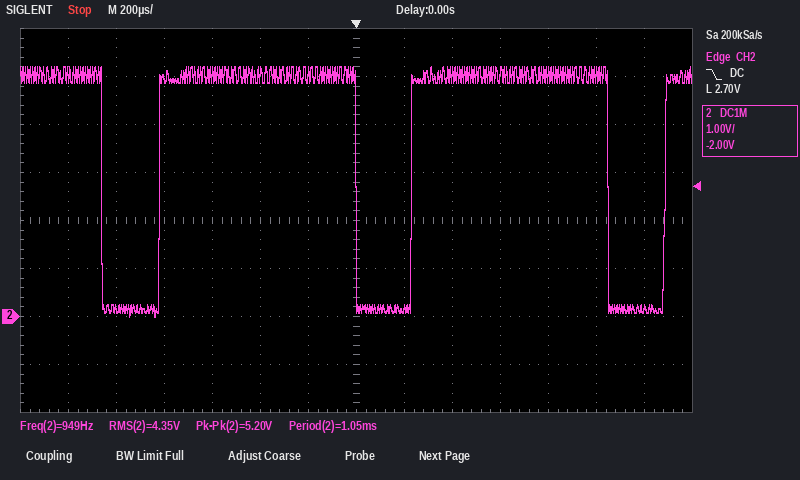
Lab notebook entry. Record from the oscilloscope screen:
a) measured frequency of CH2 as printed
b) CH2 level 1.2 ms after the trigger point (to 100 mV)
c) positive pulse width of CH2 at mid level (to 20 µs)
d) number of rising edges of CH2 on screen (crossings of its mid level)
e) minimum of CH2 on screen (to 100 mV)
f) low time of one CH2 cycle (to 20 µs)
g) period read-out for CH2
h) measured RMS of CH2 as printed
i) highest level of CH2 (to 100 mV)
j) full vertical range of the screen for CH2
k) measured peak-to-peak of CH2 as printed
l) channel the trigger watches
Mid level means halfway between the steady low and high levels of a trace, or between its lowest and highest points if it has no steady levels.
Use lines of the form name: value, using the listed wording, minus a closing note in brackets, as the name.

measured frequency of CH2 as printed: 949 Hz
CH2 level 1.2 ms after the trigger point: 200 mV
positive pulse width of CH2 at mid level: 820 µs
number of rising edges of CH2 on screen: 3
minimum of CH2 on screen: 0.0 V
low time of one CH2 cycle: 240 µs
period read-out for CH2: 1.05 ms
measured RMS of CH2 as printed: 4.35 V
highest level of CH2: 5.2 V
full vertical range of the screen for CH2: 8 V
measured peak-to-peak of CH2 as printed: 5.20 V
channel the trigger watches: CH2
